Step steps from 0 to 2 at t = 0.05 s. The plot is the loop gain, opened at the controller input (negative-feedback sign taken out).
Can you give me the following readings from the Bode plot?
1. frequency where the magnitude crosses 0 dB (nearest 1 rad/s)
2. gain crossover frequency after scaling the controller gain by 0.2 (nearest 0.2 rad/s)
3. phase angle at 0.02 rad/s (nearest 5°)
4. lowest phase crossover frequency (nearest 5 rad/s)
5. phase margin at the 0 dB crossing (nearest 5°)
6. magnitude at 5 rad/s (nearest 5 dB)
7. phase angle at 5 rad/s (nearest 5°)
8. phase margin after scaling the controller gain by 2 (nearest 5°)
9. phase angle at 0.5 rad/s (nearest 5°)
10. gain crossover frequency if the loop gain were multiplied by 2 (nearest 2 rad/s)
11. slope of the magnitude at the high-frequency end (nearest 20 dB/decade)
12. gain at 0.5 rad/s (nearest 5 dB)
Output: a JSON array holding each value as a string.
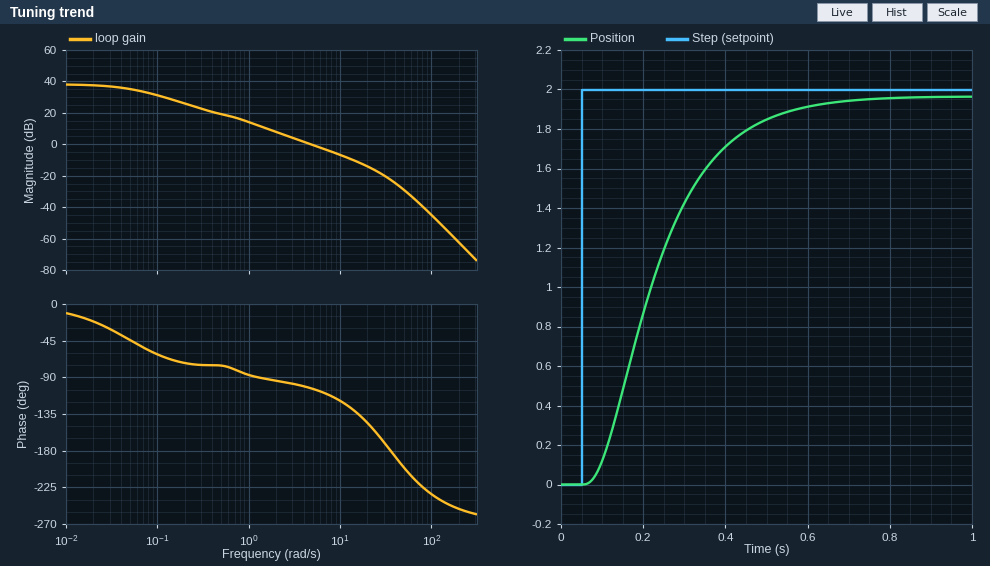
["5 rad/s", "1.0 rad/s", "-20°", "35 rad/s", "75°", "0 dB", "-105°", "65°", "-75°", "10 rad/s", "-60 dB/decade", "20 dB"]
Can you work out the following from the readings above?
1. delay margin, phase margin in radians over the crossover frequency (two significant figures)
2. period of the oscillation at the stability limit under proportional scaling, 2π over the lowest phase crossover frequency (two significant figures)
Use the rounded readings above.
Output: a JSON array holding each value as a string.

["0.26 s", "0.18 s"]
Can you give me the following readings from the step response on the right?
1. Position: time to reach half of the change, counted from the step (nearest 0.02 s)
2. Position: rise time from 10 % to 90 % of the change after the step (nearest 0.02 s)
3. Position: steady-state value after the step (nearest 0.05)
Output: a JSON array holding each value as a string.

["0.16 s", "0.32 s", "1.95"]
